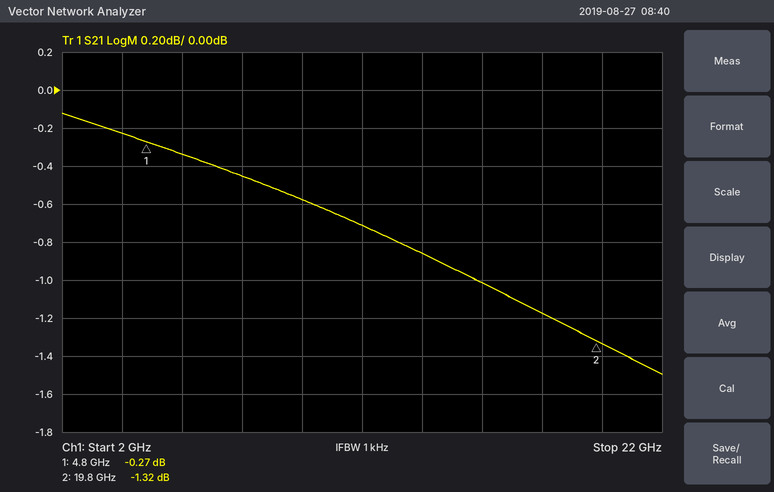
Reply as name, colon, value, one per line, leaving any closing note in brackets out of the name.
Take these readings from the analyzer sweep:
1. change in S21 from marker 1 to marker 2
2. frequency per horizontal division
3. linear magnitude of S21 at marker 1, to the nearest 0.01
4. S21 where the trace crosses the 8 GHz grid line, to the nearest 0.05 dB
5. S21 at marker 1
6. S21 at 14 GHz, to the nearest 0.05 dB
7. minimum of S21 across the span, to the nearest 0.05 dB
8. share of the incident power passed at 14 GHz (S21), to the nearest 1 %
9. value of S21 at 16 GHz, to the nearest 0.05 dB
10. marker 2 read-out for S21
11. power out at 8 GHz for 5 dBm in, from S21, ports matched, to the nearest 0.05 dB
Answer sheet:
change in S21 from marker 1 to marker 2: -1.05 dB
frequency per horizontal division: 2 GHz
linear magnitude of S21 at marker 1, to the nearest 0.01: 0.97
S21 where the trace crosses the 8 GHz grid line, to the nearest 0.05 dB: -0.45 dB
S21 at marker 1: -0.27 dB
S21 at 14 GHz, to the nearest 0.05 dB: -0.85 dB
minimum of S21 across the span, to the nearest 0.05 dB: -1.50 dB
share of the incident power passed at 14 GHz (S21), to the nearest 1 %: 82 %
value of S21 at 16 GHz, to the nearest 0.05 dB: -1.00 dB
marker 2 read-out for S21: -1.32 dB
power out at 8 GHz for 5 dBm in, from S21, ports matched, to the nearest 0.05 dB: 4.55 dBm
